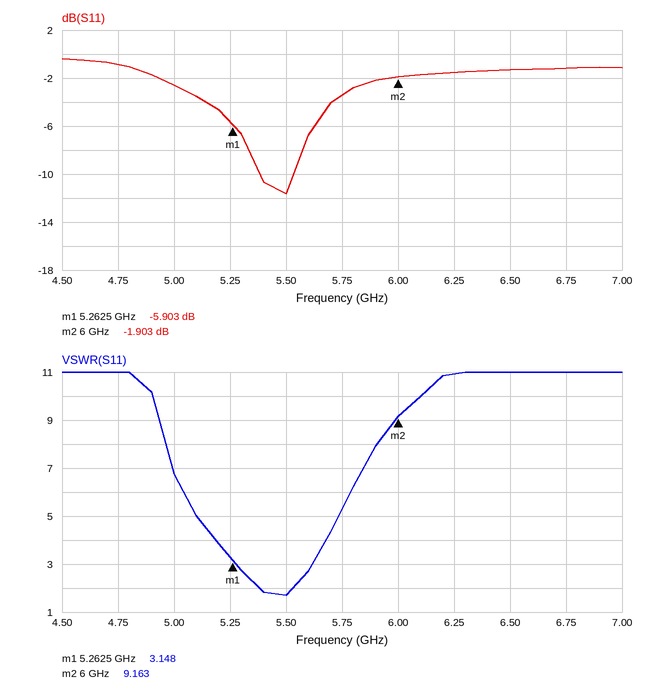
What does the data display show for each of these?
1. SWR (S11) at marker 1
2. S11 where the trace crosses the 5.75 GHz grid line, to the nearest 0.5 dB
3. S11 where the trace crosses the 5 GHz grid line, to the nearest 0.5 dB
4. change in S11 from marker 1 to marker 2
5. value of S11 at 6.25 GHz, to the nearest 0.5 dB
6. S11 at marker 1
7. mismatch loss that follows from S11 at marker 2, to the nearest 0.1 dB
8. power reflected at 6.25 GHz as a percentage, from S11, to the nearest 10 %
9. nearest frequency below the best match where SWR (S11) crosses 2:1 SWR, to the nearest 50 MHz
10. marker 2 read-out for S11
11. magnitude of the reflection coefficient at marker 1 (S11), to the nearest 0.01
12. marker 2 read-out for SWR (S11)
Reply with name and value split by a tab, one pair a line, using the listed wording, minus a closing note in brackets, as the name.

SWR (S11) at marker 1	3.148
S11 where the trace crosses the 5.75 GHz grid line, to the nearest 0.5 dB	-3.5 dB
S11 where the trace crosses the 5 GHz grid line, to the nearest 0.5 dB	-2.5 dB
change in S11 from marker 1 to marker 2	4.000 dB
value of S11 at 6.25 GHz, to the nearest 0.5 dB	-1.5 dB
S11 at marker 1	-5.903 dB
mismatch loss that follows from S11 at marker 2, to the nearest 0.1 dB	4.5 dB
power reflected at 6.25 GHz as a percentage, from S11, to the nearest 10 %	70 %
nearest frequency below the best match where SWR (S11) crosses 2:1 SWR, to the nearest 50 MHz	5.40 GHz
marker 2 read-out for S11	-1.903 dB
magnitude of the reflection coefficient at marker 1 (S11), to the nearest 0.01	0.51
marker 2 read-out for SWR	9.163
